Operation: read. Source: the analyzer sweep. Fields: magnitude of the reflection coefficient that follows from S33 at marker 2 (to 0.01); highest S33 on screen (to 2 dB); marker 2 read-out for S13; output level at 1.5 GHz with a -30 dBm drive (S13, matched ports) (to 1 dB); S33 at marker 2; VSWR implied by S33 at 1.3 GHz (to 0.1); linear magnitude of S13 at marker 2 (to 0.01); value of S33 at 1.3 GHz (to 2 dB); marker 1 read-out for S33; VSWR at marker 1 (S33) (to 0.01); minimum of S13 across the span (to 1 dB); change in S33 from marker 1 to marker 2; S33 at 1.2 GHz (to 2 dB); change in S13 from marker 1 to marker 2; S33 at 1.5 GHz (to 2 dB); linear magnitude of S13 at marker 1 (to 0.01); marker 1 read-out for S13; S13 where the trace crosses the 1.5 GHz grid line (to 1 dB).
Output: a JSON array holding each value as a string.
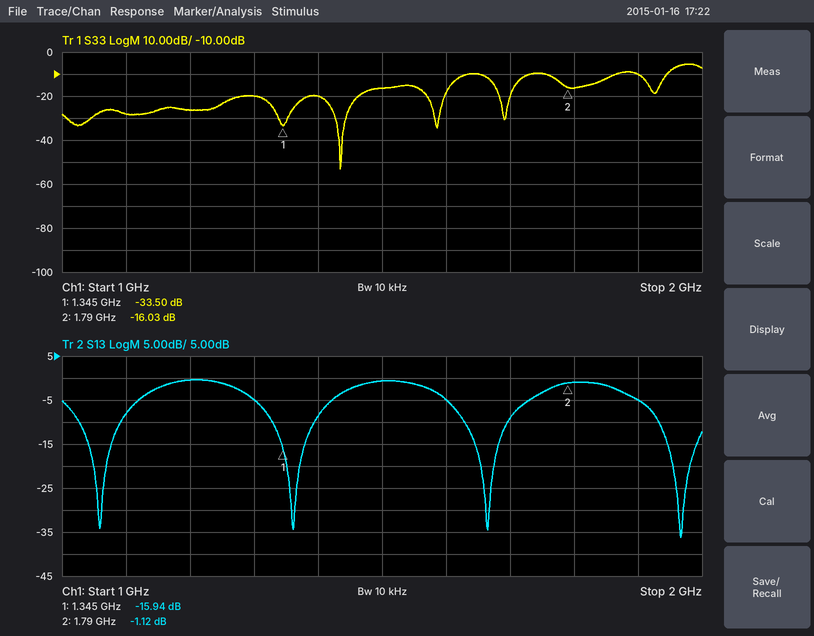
["0.16", "-6 dB", "-1.12 dB", "-31 dBm", "-16.03 dB", "1.2", "0.88", "-20 dB", "-33.50 dB", "1.04", "-36 dB", "17.47 dB", "-26 dB", "14.82 dB", "-16 dB", "0.16", "-15.94 dB", "-1 dB"]
